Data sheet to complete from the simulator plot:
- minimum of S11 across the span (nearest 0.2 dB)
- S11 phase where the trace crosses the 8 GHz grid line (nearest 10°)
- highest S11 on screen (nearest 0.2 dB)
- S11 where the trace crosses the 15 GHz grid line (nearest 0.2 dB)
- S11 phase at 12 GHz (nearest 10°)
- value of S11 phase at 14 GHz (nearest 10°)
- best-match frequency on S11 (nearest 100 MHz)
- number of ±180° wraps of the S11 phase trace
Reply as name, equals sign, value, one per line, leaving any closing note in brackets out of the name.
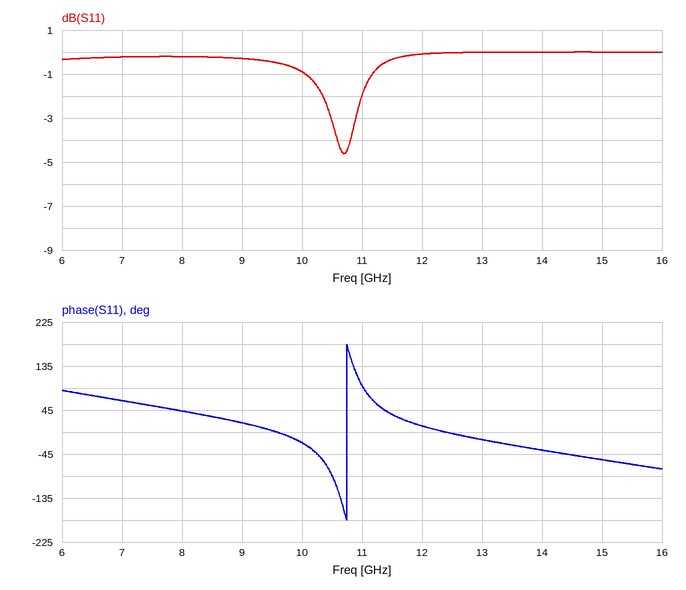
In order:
minimum of S11 across the span = -4.6 dB
S11 phase where the trace crosses the 8 GHz grid line = 40°
highest S11 on screen = 0.0 dB
S11 where the trace crosses the 15 GHz grid line = 0.0 dB
S11 phase at 12 GHz = 10°
value of S11 phase at 14 GHz = -40°
best-match frequency on S11 = 10.7 GHz
number of ±180° wraps of the S11 phase trace = 1
